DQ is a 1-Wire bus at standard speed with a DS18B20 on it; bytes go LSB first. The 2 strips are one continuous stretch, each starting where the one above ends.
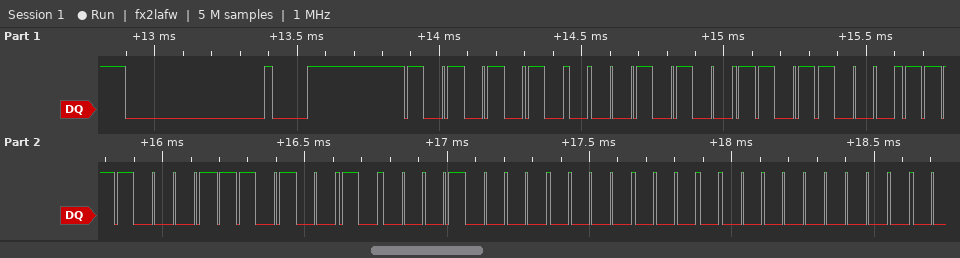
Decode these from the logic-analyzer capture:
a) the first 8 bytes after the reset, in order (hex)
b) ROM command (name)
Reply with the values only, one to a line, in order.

55 28 1B 8F 4B 08 00 00
Match ROM
